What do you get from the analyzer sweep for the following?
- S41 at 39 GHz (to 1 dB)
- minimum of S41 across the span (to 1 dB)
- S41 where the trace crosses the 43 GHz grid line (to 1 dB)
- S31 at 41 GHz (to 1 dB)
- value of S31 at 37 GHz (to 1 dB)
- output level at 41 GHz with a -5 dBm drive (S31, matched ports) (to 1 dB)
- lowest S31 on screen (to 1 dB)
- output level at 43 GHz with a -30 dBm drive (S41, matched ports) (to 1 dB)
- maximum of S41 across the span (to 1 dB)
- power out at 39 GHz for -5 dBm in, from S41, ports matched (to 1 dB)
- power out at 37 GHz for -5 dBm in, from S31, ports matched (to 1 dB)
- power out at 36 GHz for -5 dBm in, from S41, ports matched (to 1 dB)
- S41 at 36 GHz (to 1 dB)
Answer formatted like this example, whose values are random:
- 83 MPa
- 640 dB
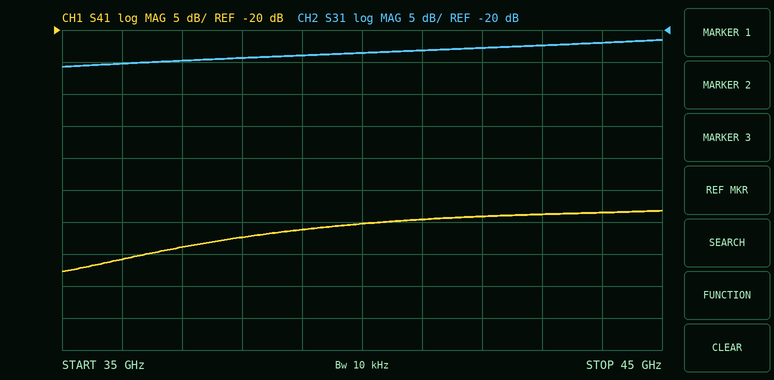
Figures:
- -51 dB
- -58 dB
- -49 dB
- -23 dB
- -25 dB
- -28 dBm
- -26 dB
- -79 dBm
- -48 dB
- -56 dBm
- -30 dBm
- -61 dBm
- -56 dB
